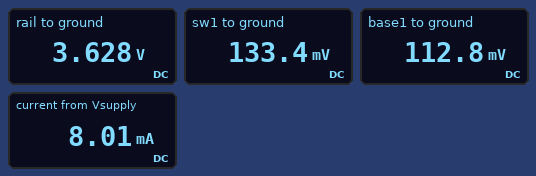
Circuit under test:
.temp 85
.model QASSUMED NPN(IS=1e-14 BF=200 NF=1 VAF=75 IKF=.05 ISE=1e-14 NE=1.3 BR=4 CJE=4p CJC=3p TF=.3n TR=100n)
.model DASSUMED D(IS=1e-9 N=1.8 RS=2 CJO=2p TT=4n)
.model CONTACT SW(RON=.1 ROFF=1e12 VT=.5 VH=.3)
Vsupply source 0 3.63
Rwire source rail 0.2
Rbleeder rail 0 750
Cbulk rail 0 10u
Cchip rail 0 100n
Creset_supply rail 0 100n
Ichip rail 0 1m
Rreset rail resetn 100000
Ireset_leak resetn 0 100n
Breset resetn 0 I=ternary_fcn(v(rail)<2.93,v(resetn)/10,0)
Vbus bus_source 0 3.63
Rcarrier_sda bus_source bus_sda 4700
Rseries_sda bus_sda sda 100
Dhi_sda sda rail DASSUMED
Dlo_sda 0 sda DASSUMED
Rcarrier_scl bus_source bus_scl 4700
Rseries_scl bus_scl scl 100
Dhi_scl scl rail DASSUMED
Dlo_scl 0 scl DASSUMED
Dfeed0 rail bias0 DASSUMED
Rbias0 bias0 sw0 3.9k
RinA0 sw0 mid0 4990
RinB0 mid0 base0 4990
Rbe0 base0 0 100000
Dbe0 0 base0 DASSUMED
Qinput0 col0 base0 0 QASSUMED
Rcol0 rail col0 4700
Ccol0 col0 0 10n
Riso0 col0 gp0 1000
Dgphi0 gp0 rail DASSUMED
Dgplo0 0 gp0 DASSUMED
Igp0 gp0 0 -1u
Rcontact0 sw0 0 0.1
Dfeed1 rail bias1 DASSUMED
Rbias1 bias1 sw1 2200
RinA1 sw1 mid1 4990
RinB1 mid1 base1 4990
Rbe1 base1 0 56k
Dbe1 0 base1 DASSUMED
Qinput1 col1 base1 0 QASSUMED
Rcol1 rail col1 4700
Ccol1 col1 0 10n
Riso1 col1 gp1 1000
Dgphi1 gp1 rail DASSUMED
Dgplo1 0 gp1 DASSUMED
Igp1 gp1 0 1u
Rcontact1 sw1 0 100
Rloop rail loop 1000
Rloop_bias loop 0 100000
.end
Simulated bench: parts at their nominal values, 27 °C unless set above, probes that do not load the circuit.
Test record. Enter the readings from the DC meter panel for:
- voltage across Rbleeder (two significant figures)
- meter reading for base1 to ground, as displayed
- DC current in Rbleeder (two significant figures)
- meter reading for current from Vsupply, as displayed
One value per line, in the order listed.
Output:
3.6 V
112.8 mV
4.8 mA
8.01 mA
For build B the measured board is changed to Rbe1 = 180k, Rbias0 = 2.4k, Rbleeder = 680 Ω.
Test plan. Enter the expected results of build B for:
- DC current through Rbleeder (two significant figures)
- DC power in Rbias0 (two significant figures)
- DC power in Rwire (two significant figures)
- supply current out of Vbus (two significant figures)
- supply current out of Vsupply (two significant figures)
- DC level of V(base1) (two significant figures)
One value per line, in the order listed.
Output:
5.3 mA
3.9 mW
16 µW
130 nA
9.0 mA
130 mV
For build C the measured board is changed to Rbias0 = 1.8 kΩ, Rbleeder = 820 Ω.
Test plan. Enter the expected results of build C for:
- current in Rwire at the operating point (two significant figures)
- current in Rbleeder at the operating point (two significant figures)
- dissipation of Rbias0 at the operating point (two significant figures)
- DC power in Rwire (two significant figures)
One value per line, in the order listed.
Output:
8.5 mA
4.4 mA
5.2 mW
14 µW
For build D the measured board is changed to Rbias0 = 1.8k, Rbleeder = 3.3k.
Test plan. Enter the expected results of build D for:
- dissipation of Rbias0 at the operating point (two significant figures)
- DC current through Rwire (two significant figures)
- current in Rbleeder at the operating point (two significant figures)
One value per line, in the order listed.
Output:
5.2 mW
5.2 mA
1.1 mA
